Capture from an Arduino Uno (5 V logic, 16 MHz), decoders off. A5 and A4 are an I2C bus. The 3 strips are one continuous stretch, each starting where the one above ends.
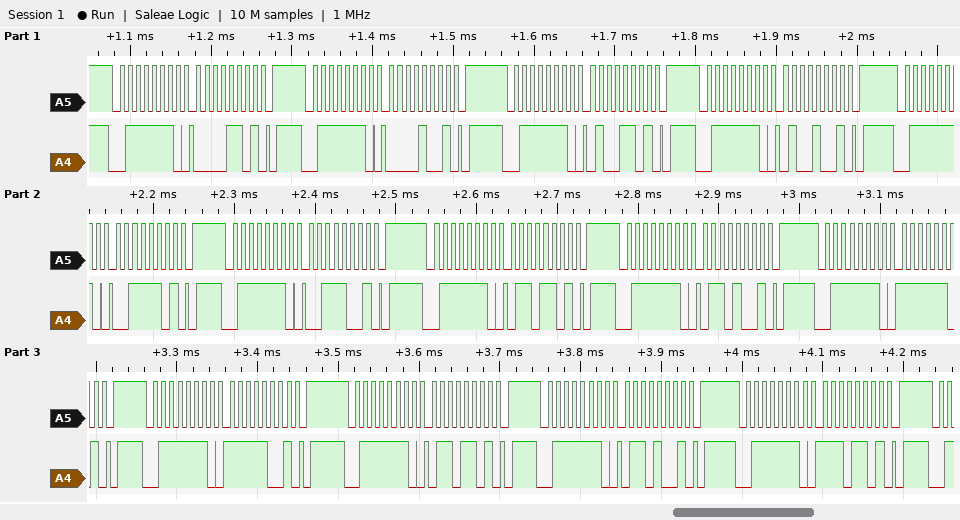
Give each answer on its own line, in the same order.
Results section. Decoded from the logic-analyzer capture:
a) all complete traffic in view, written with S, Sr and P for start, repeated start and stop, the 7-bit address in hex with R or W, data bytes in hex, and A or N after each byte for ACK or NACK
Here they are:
S 3FW A 0D A P S 3FW A 09 A P S 3FW A 4D A P S 3FW A 49 A P S 3FW A 3D A P S 3FW A 39 A P S 3FW A 6D A P S 3FW A 69 A P S 3FW A FD A P S 3FW A F9 A P S 3FW A 6D A P S 3FW A 69 A P S 3FW A ED A P
